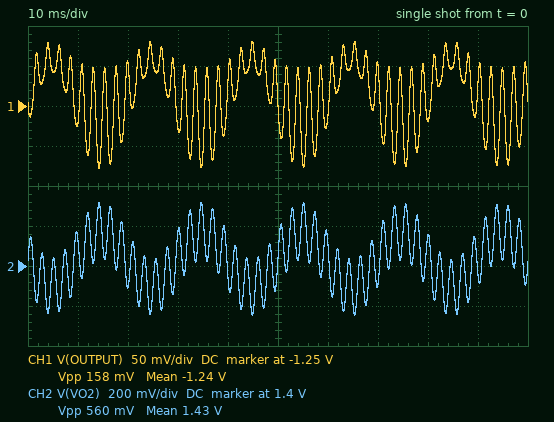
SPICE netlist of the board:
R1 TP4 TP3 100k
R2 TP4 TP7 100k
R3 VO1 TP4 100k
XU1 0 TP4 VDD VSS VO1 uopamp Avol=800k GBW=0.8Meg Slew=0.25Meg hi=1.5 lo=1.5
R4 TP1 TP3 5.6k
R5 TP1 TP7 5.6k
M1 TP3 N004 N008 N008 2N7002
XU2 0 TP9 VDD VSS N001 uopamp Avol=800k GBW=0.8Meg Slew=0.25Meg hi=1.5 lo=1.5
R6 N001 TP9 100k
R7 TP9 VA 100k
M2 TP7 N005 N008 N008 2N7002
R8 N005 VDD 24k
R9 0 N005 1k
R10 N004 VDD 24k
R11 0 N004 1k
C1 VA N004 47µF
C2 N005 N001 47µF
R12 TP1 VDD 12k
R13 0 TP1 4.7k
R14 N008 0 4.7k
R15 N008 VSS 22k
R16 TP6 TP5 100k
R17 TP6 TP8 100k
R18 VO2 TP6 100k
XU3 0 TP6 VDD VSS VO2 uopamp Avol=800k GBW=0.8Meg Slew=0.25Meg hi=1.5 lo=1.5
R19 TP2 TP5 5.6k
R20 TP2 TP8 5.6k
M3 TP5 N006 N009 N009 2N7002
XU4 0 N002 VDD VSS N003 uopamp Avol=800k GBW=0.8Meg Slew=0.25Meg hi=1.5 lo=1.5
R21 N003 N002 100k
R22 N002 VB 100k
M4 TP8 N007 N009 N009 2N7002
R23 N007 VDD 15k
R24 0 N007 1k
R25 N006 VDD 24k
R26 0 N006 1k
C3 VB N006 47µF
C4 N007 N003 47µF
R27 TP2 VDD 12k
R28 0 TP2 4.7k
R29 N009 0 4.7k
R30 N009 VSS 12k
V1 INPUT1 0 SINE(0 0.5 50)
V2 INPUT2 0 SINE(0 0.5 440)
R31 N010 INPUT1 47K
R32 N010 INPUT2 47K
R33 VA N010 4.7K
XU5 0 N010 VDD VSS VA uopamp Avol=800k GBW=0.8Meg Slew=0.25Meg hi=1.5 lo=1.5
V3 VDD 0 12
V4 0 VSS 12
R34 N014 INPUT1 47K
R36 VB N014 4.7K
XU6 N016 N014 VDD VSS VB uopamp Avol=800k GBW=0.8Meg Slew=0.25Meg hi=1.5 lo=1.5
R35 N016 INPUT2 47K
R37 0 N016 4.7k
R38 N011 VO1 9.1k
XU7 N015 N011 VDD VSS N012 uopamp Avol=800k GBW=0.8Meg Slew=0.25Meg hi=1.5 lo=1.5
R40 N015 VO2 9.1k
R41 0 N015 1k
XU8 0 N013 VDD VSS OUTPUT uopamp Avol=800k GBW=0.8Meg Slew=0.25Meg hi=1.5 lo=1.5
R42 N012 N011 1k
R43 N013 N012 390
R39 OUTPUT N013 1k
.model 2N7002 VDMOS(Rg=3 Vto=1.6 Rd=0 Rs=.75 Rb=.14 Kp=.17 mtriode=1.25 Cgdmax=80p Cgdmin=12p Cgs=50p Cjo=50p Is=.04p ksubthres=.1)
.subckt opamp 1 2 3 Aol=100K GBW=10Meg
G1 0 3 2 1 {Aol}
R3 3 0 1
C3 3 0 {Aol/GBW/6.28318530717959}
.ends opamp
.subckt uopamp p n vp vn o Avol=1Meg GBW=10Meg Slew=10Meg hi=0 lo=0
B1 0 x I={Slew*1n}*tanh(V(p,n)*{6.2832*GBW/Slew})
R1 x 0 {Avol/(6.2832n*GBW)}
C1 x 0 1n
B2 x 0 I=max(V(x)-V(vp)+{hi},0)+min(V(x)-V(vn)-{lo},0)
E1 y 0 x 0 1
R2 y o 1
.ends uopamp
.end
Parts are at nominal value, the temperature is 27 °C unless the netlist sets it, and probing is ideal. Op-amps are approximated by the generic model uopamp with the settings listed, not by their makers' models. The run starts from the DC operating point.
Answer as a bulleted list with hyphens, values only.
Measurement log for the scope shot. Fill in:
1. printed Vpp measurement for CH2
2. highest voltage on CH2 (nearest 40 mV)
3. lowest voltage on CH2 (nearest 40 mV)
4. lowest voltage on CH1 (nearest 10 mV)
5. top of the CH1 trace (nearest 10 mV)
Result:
- 560 mV
- 1.72 V
- 1.16 V
- -1.33 V
- -1.17 V
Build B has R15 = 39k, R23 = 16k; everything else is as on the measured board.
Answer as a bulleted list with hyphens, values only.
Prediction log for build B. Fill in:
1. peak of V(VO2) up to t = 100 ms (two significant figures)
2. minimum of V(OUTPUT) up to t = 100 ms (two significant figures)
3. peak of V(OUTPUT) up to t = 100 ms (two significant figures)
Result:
- 1.7 V
- -1.9 V
- -1.8 V
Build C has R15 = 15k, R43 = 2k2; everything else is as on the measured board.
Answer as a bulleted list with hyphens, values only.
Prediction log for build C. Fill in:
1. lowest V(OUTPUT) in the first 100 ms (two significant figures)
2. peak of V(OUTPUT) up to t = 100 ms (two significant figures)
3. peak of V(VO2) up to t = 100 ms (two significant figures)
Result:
- -110 mV
- -85 mV
- 1.7 V
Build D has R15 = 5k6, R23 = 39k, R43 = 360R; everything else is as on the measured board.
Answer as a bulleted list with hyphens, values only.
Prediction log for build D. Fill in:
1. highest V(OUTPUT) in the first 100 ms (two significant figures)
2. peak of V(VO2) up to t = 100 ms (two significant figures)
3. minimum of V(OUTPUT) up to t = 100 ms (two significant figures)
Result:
- 1.5 V
- 1.1 V
- 1.4 V
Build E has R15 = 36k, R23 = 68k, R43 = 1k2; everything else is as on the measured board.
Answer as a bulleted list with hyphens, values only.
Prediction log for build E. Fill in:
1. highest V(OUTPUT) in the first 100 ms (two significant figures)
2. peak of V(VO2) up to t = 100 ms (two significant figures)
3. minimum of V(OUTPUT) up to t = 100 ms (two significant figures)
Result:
- -490 mV
- 860 mV
- -530 mV
